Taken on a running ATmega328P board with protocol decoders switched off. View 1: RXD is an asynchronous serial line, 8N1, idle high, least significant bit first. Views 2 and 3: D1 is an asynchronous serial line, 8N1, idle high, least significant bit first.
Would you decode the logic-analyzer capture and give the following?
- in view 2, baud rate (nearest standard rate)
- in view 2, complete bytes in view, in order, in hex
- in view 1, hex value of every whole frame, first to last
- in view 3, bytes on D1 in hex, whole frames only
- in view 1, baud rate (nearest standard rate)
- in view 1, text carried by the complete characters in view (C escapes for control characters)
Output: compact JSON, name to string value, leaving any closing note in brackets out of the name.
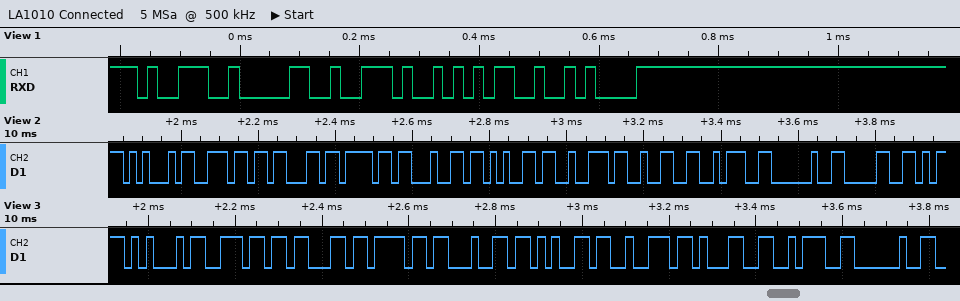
{"in view 2, baud rate": "57600 baud", "in view 2, complete bytes in view, in order, in hex": "0x45 0x6E 0x63 0x6F 0x64 0x65 0x72 0x32 0x3A 0x20 0x30", "in view 1, hex value of every whole frame, first to last": "39 30 2E 35 0A", "in view 3, bytes on D1 in hex, whole frames only": "45 6E 63 6F 64 65 72 31 3A 20", "in view 1, baud rate": "57600 baud", "in view 1, text carried by the complete characters in view": "\"90.5\\n\""}
